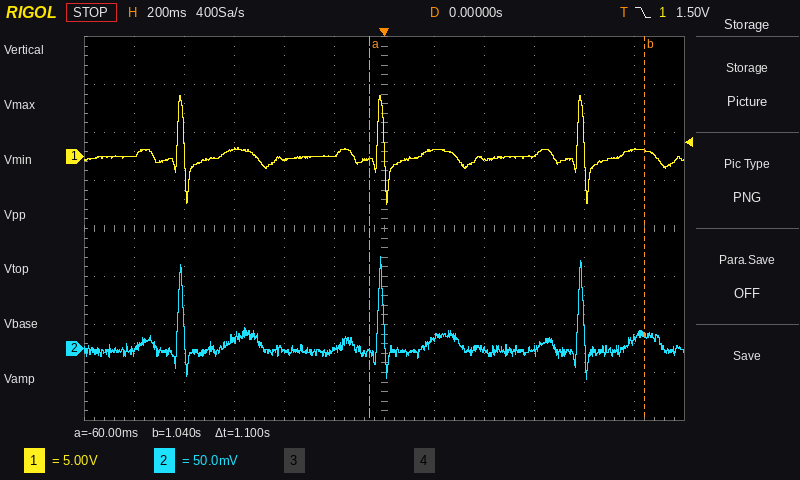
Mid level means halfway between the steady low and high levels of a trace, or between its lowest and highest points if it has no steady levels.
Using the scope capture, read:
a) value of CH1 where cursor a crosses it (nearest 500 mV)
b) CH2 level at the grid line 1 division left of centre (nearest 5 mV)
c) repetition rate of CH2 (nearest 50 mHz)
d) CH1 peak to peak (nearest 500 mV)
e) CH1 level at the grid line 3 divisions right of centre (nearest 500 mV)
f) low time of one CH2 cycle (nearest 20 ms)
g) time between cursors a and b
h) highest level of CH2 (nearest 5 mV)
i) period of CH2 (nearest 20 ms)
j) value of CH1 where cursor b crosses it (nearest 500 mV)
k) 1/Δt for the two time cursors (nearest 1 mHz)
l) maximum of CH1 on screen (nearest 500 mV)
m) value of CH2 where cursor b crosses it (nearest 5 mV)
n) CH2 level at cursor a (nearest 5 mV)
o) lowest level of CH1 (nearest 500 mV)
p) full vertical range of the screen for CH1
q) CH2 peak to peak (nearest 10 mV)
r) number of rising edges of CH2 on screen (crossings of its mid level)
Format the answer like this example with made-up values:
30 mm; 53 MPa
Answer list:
-500 mV; 0 mV; 1.25 Hz; 11.5 V; 0.0 V; 780 ms; 1.1 s; 95 mV; 800 ms; 500 mV; 909 mHz; 6.5 V; 15 mV; -5 mV; -5.0 V; 40 V; 130 mV; 3
